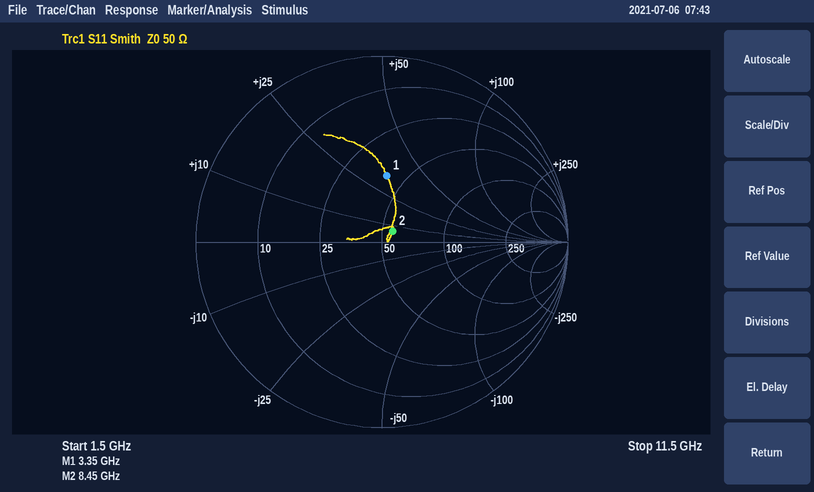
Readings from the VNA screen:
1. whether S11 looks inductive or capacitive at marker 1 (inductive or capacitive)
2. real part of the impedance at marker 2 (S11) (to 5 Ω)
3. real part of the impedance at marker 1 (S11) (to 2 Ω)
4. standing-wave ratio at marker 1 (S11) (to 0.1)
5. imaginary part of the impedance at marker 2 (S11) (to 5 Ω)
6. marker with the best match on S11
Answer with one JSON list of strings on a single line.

["inductive", "55 Ω", "40 Ω", "2.1", "+5 Ω", "marker 2"]
